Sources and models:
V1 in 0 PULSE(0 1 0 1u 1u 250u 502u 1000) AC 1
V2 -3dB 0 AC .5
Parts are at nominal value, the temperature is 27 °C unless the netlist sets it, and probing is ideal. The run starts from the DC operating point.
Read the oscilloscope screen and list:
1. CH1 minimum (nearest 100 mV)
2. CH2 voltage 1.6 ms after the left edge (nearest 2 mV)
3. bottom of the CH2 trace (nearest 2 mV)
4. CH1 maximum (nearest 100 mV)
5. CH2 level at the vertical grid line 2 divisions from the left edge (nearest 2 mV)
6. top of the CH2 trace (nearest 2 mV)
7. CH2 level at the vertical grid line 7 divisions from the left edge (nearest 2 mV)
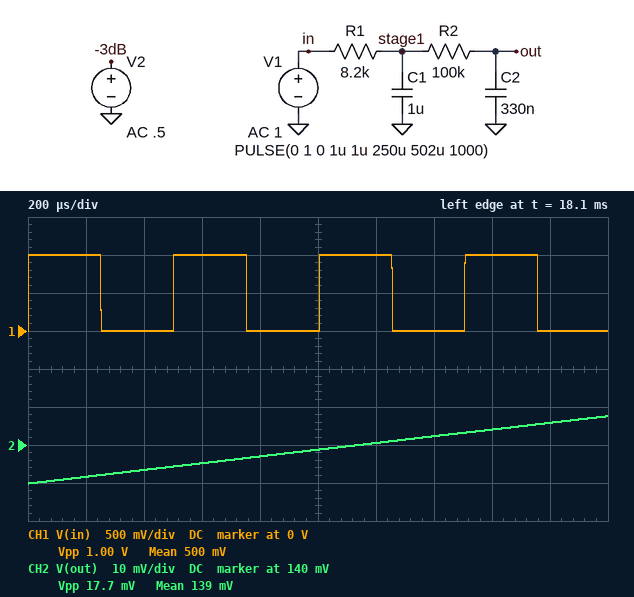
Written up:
0 V
144 mV
130 mV
1.0 V
134 mV
148 mV
142 mV
